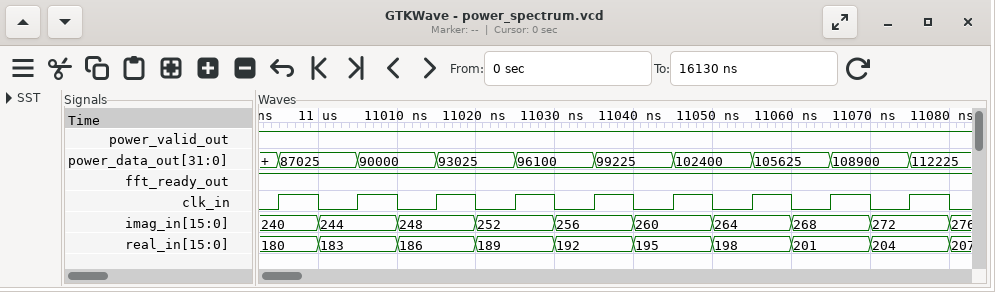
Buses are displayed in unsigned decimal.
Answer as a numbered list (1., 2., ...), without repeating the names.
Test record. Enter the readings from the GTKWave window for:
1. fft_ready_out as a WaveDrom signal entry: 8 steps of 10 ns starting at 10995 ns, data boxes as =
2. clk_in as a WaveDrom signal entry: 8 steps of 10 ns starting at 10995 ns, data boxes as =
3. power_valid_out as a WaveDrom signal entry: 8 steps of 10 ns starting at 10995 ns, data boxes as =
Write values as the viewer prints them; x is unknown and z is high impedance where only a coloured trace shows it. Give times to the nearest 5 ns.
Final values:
1. {name: 'fft_ready_out', wave: '1.......'}
2. {name: 'clk_in', wave: 'p.......'}
3. {name: 'power_valid_out', wave: '1.......'}
